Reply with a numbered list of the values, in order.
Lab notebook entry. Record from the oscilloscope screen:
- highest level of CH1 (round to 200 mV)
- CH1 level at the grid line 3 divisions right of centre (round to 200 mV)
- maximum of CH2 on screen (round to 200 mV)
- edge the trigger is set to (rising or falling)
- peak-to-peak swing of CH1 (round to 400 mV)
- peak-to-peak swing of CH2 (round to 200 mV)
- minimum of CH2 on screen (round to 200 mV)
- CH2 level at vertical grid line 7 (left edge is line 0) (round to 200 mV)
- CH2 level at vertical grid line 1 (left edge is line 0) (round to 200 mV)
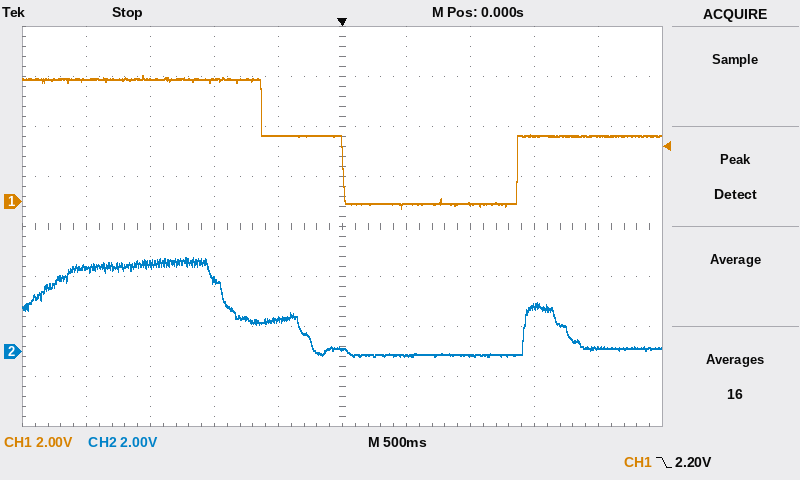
1. 5.0 V
2. 2.6 V
3. 3.8 V
4. falling
5. 5.2 V
6. 4.0 V
7. -200 mV
8. -200 mV
9. 3.4 V
